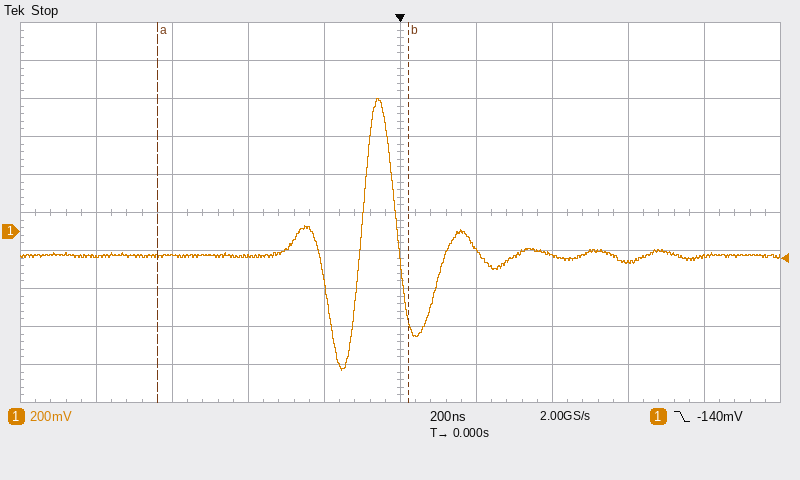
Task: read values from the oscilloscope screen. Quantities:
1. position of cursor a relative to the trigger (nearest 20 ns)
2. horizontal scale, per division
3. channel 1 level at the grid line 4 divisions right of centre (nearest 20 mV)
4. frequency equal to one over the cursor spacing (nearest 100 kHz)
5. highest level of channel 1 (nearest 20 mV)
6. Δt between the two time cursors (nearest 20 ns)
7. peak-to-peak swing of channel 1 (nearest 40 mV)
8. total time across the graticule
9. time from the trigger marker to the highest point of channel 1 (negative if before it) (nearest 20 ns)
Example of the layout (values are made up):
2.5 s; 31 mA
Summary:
-640 ns; 200 ns; -140 mV; 1.5 MHz; 700 mV; 660 ns; 1.44 V; 2 µs; -60 ns
